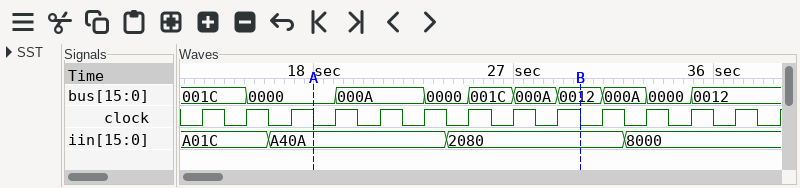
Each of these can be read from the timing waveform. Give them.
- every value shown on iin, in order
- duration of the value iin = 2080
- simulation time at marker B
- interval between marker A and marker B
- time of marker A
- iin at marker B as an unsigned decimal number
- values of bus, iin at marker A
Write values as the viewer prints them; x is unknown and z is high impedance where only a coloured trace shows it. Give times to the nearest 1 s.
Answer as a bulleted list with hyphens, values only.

- A01C, A40A, 2080, 8000
- 8 s
- 30 s
- 12 s
- 18 s
- 8320
- bus=0000, iin=A40A
